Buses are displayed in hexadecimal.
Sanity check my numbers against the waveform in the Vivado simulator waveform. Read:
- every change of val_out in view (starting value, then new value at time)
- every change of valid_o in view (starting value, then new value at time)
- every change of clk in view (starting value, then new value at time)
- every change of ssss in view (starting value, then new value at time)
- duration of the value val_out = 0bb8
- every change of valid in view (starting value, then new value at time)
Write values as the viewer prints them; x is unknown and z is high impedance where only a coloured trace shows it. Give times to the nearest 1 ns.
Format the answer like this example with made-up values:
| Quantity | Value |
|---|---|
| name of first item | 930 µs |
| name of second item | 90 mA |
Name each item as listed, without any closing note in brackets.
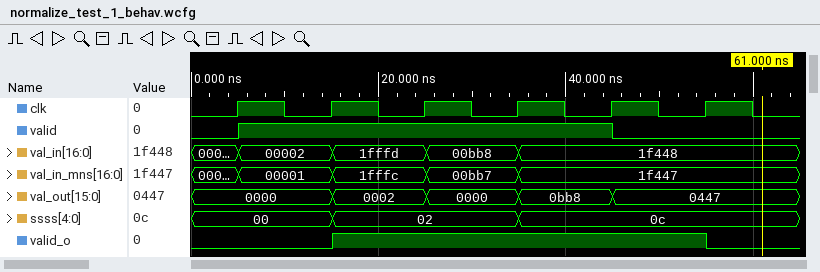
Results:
| Quantity | Value |
|---|---|
| every change of val_out in view | 0000, 0002 at 15 ns, 0000 at 25 ns, 0bb8 at 35 ns, 0447 at 45 ns |
| every change of valid_o in view | 0, 1 at 15 ns, 0 at 55 ns |
| every change of clk in view | 0, 1 at 5 ns, 0 at 10 ns, 1 at 15 ns, 0 at 20 ns, 1 at 25 ns, 0 at 30 ns, 1 at 35 ns, 0 at 40 ns, 1 at 45 ns, 0 at 50 ns, 1 at 55 ns, 0 at 60 ns |
| every change of ssss in view | 00, 02 at 15 ns, 0c at 35 ns |
| duration of the value val_out = 0bb8 | 10 ns |
| every change of valid in view | 0, 1 at 5 ns, 0 at 45 ns |
